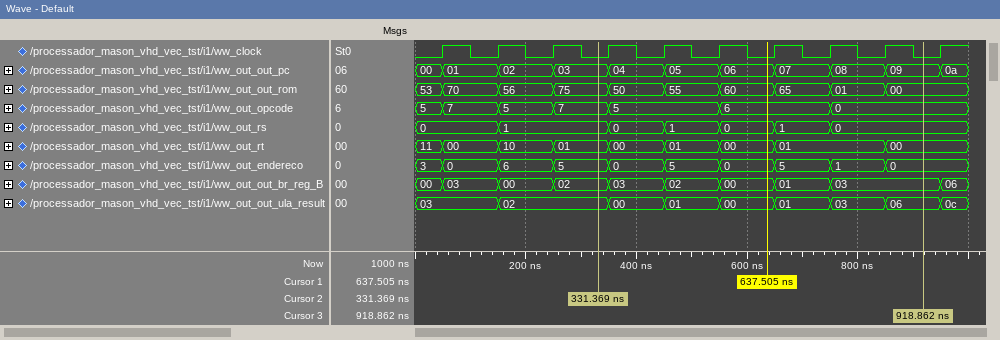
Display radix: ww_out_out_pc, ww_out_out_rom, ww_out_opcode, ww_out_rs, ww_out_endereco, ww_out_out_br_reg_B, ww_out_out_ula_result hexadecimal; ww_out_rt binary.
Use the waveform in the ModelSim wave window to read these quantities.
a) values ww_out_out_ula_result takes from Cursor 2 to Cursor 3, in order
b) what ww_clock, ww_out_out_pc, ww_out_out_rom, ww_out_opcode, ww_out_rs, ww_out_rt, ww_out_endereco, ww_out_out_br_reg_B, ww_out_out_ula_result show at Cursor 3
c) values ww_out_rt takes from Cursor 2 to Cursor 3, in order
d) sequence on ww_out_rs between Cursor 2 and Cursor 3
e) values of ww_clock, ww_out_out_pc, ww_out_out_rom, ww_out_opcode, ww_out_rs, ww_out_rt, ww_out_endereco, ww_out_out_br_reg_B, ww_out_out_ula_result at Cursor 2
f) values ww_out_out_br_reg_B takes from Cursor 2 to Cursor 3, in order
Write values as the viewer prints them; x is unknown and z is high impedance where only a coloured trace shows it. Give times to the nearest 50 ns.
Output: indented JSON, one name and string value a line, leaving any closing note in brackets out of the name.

{
  "values ww_out_out_ula_result takes from Cursor 2 to Cursor 3, in order": "02, 00, 01, 00, 01, 03, 06",
  "what ww_clock, ww_out_out_pc, ww_out_out_rom, ww_out_opcode, ww_out_rs, ww_out_rt, ww_out_endereco, ww_out_out_br_reg_B, ww_out_out_ula_result show at Cursor 3": "ww_clock=0, ww_out_out_pc=09, ww_out_out_rom=00, ww_out_opcode=0, ww_out_rs=0, ww_out_rt=00, ww_out_endereco=0, ww_out_out_br_reg_B=03, ww_out_out_ula_result=06",
  "values ww_out_rt takes from Cursor 2 to Cursor 3, in order": "01, 00, 01, 00, 01, 00",
  "sequence on ww_out_rs between Cursor 2 and Cursor 3": "1, 0, 1, 0, 1, 0",
  "values of ww_clock, ww_out_out_pc, ww_out_out_rom, ww_out_opcode, ww_out_rs, ww_out_rt, ww_out_endereco, ww_out_out_br_reg_B, ww_out_out_ula_result at Cursor 2": "ww_clock=0, ww_out_out_pc=03, ww_out_out_rom=75, ww_out_opcode=7, ww_out_rs=1, ww_out_rt=01, ww_out_endereco=5, ww_out_out_br_reg_B=02, ww_out_out_ula_result=02",
  "values ww_out_out_br_reg_B takes from Cursor 2 to Cursor 3, in order": "02, 03, 02, 00, 01, 03"
}
